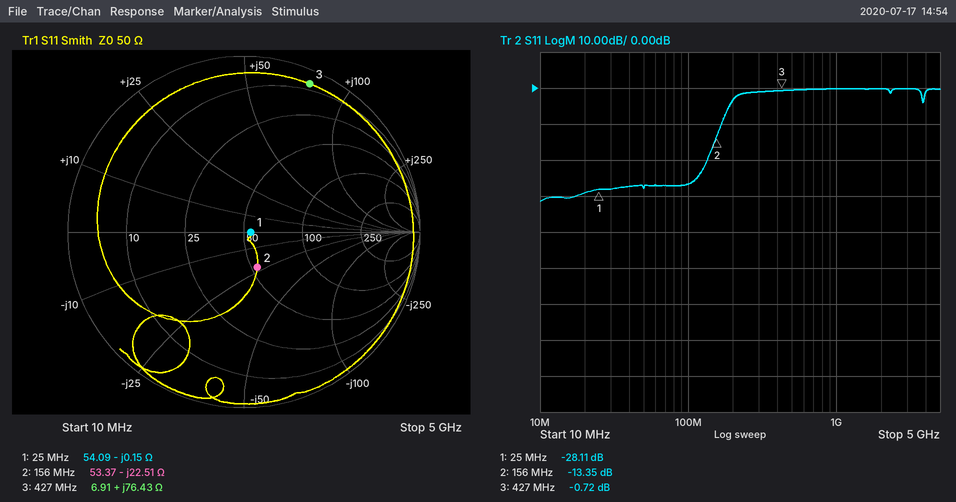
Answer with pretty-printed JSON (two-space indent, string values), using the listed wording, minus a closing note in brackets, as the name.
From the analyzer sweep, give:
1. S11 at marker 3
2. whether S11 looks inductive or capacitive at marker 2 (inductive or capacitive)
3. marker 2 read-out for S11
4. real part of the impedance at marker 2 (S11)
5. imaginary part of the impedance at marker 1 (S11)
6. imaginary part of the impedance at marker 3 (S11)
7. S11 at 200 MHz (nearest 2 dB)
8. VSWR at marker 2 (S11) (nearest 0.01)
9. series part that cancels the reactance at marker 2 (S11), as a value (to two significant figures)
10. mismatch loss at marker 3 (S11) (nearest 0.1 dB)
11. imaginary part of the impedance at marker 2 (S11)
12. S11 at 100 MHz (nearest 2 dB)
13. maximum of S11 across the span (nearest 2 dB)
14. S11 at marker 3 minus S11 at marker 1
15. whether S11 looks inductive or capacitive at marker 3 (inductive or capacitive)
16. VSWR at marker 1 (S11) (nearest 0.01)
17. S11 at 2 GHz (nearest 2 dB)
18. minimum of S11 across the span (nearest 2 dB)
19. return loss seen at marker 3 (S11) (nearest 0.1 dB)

{
  "S11 at marker 3": "-0.72 dB",
  "whether S11 looks inductive or capacitive at marker 2": "capacitive",
  "marker 2 read-out for S11": "-13.35 dB",
  "real part of the impedance at marker 2": "53.37 Ω",
  "imaginary part of the impedance at marker 1": "-0.15 Ω",
  "imaginary part of the impedance at marker 3": "+76.43 Ω",
  "S11 at 200 MHz": "-4 dB",
  "VSWR at marker 2 (S11)": "1.55",
  "series part that cancels the reactance at marker 2 (S11), as a value": "23 nH",
  "mismatch loss at marker 3 (S11)": "8.2 dB",
  "imaginary part of the impedance at marker 2": "-22.51 Ω",
  "S11 at 100 MHz": "-26 dB",
  "maximum of S11 across the span": "0 dB",
  "S11 at marker 3 minus S11 at marker 1": "27.39 dB",
  "whether S11 looks inductive or capacitive at marker 3": "inductive",
  "VSWR at marker 1 (S11)": "1.08",
  "S11 at 2 GHz": "0 dB",
  "minimum of S11 across the span": "-32 dB",
  "return loss seen at marker 3 (S11)": "0.7 dB"
}
